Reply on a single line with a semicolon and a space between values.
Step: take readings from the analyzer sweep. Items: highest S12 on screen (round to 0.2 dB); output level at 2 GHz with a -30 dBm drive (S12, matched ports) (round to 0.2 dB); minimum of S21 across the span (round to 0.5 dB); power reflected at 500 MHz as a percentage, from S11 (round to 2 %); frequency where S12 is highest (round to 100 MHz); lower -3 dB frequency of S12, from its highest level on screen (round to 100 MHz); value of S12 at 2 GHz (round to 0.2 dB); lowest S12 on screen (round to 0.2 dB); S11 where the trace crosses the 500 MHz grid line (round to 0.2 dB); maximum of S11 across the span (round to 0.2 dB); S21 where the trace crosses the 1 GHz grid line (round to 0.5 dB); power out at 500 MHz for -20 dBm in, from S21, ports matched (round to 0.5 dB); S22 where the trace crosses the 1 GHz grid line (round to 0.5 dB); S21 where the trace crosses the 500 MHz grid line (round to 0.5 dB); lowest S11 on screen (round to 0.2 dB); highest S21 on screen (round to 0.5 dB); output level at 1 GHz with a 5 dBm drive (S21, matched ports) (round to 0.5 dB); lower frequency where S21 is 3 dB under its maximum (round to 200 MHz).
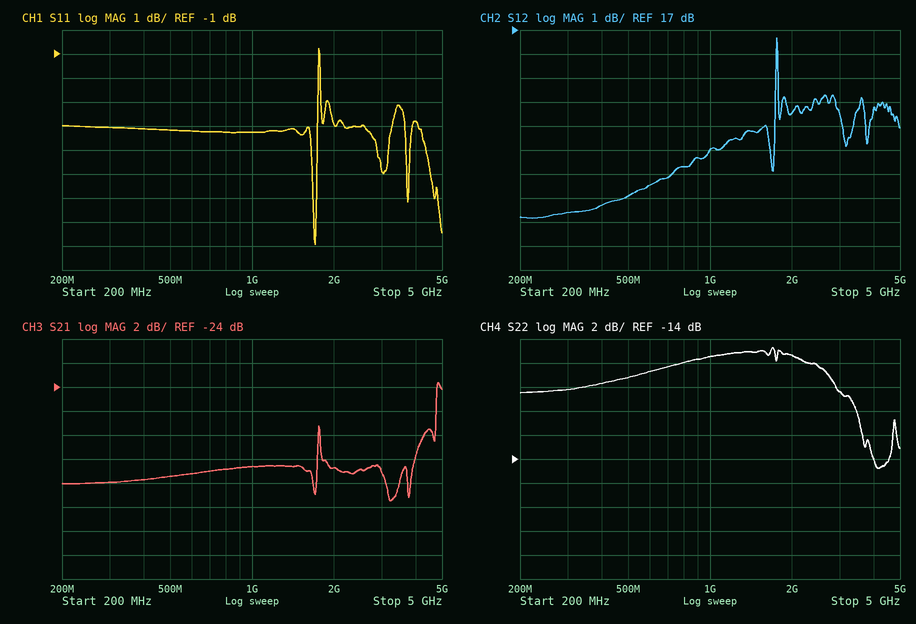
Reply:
16.6 dB; -16.4 dBm; -33.5 dB; 38 %; 1.8 GHz; 1.7 GHz; 13.6 dB; 9.2 dB; -4.2 dB; -0.8 dB; -30.5 dB; -51.5 dBm; -5.5 dB; -31.5 dB; -9.0 dB; -23.5 dB; -25.5 dBm; 4.8 GHz
